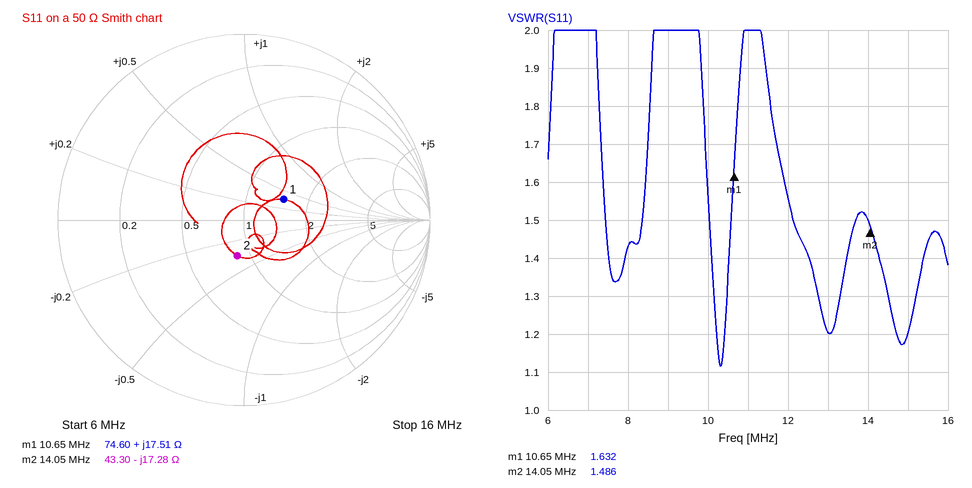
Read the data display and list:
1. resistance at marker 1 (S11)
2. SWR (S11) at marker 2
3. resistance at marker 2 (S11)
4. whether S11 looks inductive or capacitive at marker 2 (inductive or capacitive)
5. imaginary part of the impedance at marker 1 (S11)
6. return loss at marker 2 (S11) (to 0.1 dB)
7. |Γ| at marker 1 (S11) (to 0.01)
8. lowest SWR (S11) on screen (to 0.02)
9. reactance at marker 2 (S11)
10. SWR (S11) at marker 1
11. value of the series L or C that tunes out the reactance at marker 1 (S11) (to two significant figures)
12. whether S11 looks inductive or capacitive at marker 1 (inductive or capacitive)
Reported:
74.60 Ω
1.486
43.30 Ω
capacitive
+17.51 Ω
14.2 dB
0.24
1.12
-17.28 Ω
1.632
850 pF
inductive
